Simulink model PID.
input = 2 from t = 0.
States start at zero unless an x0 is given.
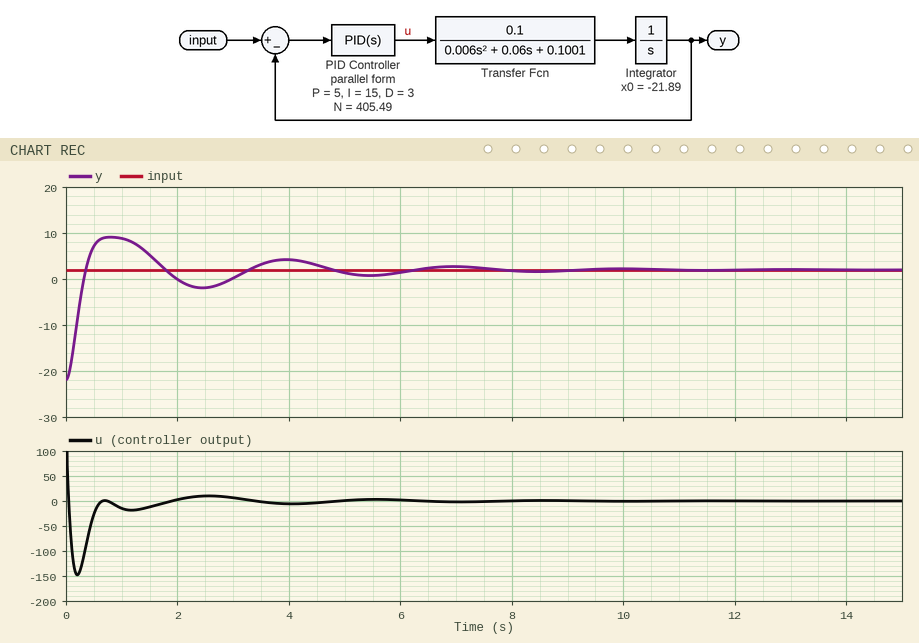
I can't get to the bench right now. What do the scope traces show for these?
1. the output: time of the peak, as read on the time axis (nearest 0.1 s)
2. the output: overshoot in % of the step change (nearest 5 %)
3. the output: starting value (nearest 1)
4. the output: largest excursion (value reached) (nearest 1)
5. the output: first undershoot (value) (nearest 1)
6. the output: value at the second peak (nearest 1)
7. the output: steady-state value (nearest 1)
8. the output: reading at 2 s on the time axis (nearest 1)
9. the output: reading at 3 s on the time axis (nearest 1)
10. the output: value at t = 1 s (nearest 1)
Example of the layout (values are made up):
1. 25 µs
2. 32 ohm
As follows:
1. 0.8 s
2. 30 %
3. -22
4. 9
5. -2
6. 4
7. 2
8. 0
9. 0
10. 9
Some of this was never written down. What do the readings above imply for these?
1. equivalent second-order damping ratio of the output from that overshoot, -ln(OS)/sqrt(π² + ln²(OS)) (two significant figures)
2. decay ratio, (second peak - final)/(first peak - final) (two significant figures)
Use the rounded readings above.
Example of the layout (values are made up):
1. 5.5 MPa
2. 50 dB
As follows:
1. 0.36
2. 0.29
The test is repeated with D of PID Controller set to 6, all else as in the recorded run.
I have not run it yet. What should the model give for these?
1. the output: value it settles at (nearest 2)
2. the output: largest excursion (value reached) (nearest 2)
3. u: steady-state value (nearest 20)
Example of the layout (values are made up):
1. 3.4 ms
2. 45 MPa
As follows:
1. 2
2. 6
3. 0
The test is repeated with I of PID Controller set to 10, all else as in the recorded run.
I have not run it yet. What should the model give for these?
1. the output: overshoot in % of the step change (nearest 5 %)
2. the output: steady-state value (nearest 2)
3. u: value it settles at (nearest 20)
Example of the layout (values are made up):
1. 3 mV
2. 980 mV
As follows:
1. 20 %
2. 2
3. 0
